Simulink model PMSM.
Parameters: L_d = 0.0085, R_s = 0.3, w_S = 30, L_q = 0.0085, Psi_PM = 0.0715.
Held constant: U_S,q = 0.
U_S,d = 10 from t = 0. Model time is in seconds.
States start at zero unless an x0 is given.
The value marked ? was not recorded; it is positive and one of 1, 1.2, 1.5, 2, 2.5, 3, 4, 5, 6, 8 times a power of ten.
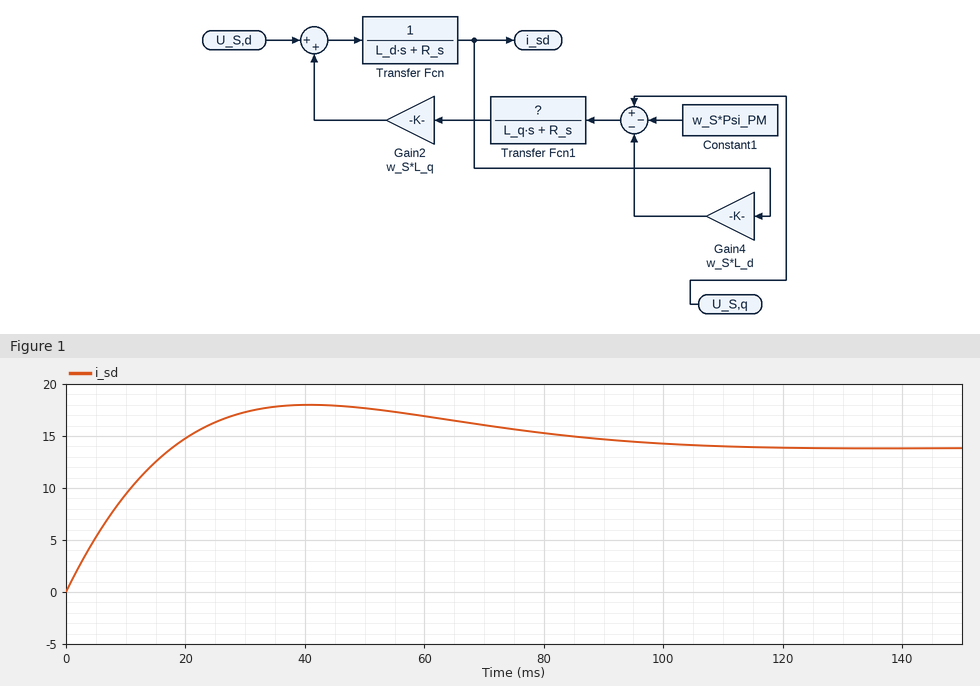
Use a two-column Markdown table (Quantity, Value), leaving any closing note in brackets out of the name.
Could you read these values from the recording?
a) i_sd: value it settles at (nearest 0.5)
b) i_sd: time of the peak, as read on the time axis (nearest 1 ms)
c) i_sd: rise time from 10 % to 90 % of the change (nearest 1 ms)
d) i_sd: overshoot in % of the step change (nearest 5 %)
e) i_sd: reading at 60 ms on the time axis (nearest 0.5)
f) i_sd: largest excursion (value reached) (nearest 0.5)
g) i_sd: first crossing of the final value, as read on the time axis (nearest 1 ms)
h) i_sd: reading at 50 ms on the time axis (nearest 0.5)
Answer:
| Quantity | Value |
|---|---|
| i_sd: value it settles at | 14.0 |
| i_sd: time of the peak, as read on the time axis | 41 ms |
| i_sd: rise time from 10 % to 90 % of the change | 14 ms |
| i_sd: overshoot in % of the step change | 30 % |
| i_sd: reading at 60 ms on the time axis | 17.0 |
| i_sd: largest excursion (value reached) | 18.0 |
| i_sd: first crossing of the final value, as read on the time axis | 18 ms |
| i_sd: reading at 50 ms on the time axis | 17.5 |
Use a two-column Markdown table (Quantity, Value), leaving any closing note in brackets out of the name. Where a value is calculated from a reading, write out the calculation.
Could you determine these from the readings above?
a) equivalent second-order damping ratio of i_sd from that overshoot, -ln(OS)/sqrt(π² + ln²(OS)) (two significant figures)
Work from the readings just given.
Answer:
| Quantity | Value |
|---|---|
| equivalent second-order damping ratio of i_sd from that overshoot, -ln(OS)/sqrt(π² + ln²(OS)) | ln(0.3) = -1.204; 1.204 / sqrt(9.870 + 1.450) = 0.36 |
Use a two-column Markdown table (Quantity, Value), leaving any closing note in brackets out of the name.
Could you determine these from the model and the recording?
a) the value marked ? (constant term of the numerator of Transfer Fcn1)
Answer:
| Quantity | Value |
|---|---|
| the value marked ? | 1.2 |
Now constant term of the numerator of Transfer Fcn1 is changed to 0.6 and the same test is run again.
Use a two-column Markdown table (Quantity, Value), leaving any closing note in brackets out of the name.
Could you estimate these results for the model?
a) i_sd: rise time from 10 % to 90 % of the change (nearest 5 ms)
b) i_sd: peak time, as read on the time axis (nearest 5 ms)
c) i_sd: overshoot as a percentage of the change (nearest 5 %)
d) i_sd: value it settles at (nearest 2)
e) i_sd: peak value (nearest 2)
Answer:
| Quantity | Value |
|---|---|
| i_sd: rise time from 10 % to 90 % of the change | 25 ms |
| i_sd: peak time, as read on the time axis | 60 ms |
| i_sd: overshoot as a percentage of the change | 10 % |
| i_sd: value it settles at | 20 |
| i_sd: peak value | 22 |
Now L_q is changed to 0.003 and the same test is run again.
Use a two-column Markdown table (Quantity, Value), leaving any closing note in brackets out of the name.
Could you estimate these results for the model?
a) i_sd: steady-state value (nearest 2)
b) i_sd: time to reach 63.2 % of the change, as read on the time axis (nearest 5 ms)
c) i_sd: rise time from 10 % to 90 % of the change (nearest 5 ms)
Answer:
| Quantity | Value |
|---|---|
| i_sd: steady-state value | 24 |
| i_sd: time to reach 63.2 % of the change, as read on the time axis | 20 ms |
| i_sd: rise time from 10 % to 90 % of the change | 40 ms |
